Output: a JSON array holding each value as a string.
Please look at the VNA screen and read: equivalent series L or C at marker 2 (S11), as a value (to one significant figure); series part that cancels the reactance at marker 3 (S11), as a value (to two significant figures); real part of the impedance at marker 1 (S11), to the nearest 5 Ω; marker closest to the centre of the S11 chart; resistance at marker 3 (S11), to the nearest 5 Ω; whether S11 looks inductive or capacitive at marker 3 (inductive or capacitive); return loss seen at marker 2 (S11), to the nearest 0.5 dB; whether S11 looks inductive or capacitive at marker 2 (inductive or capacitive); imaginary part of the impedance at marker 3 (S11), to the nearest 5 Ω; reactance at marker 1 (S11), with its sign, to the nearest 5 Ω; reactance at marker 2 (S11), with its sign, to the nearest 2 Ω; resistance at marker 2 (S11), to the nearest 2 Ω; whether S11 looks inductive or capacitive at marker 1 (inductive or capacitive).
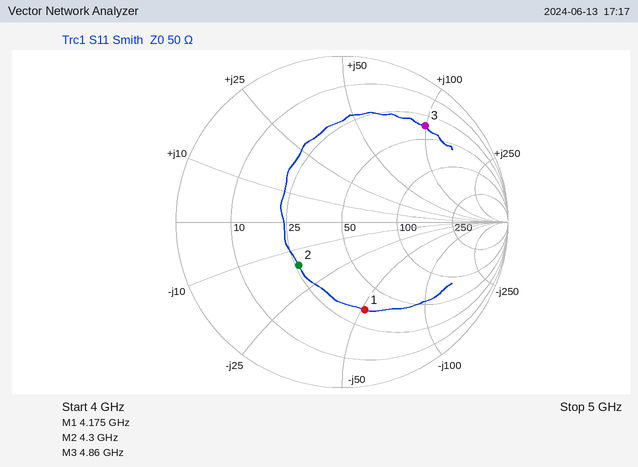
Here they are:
["2 pF", "330 fF", "35 Ω", "marker 2", "35 Ω", "inductive", "8.5 dB", "capacitive", "+100 Ω", "-50 Ω", "-16 Ω", "26 Ω", "capacitive"]
